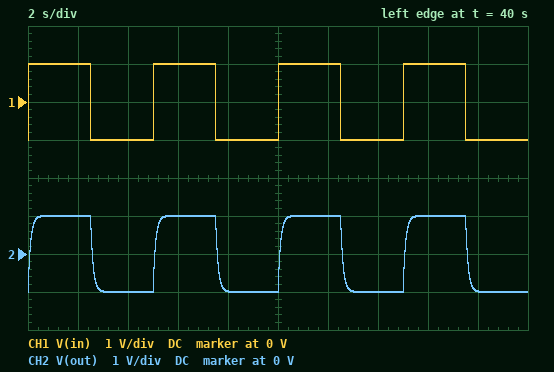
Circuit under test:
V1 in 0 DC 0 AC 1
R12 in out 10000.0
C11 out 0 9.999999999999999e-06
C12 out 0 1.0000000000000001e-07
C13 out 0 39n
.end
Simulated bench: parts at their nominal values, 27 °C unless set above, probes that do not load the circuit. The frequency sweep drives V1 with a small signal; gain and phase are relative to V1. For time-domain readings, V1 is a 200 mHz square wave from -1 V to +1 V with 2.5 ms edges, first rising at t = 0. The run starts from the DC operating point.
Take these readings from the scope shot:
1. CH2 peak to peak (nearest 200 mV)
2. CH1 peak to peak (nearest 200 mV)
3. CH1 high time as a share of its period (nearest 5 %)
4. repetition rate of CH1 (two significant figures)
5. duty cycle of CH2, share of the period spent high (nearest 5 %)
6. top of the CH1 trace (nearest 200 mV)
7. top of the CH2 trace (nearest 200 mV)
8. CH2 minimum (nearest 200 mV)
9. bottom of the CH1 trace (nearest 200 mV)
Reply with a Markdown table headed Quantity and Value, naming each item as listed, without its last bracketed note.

| Quantity | Value |
|---|---|
| CH2 peak to peak | 2.0 V |
| CH1 peak to peak | 2.0 V |
| CH1 high time as a share of its period | 50 % |
| repetition rate of CH1 | 200 mHz |
| duty cycle of CH2, share of the period spent high | 50 % |
| top of the CH1 trace | 1.0 V |
| top of the CH2 trace | 1.0 V |
| CH2 minimum | -1.0 V |
| bottom of the CH1 trace | -1.0 V |
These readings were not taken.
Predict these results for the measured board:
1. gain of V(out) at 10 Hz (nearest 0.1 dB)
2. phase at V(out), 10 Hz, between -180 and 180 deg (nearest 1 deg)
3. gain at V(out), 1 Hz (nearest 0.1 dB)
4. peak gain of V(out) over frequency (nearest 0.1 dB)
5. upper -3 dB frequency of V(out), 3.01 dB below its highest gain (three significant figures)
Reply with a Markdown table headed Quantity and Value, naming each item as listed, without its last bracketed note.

| Quantity | Value |
|---|---|
| gain of V(out) at 10 Hz | -16.2 dB |
| phase at V(out), 10 Hz, between -180 and 180 deg | -81 deg |
| gain at V(out), 1 Hz | -1.5 dB |
| peak gain of V(out) over frequency | 0 dB |
| upper -3 dB frequency of V(out), 3.01 dB below its highest gain | 1.57 Hz |
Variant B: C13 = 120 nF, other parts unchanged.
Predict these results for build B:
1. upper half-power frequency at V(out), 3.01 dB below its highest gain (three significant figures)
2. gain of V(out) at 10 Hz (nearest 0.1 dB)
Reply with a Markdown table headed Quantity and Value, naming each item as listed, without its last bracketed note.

| Quantity | Value |
|---|---|
| upper half-power frequency at V(out), 3.01 dB below its highest gain | 1.56 Hz |
| gain of V(out) at 10 Hz | -16.3 dB |
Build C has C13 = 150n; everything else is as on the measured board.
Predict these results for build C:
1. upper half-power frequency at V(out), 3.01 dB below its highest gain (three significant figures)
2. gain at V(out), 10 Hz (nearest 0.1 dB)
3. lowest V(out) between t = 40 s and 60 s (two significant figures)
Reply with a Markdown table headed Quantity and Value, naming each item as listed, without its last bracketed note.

| Quantity | Value |
|---|---|
| upper half-power frequency at V(out), 3.01 dB below its highest gain | 1.55 Hz |
| gain at V(out), 10 Hz | -16.3 dB |
| lowest V(out) between t = 40 s and 60 s | -1.0 V |
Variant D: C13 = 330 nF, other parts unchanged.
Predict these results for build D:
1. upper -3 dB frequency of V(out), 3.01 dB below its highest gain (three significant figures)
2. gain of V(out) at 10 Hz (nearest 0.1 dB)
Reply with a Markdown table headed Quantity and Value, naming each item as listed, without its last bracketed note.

| Quantity | Value |
|---|---|
| upper -3 dB frequency of V(out), 3.01 dB below its highest gain | 1.53 Hz |
| gain of V(out) at 10 Hz | -16.4 dB |
